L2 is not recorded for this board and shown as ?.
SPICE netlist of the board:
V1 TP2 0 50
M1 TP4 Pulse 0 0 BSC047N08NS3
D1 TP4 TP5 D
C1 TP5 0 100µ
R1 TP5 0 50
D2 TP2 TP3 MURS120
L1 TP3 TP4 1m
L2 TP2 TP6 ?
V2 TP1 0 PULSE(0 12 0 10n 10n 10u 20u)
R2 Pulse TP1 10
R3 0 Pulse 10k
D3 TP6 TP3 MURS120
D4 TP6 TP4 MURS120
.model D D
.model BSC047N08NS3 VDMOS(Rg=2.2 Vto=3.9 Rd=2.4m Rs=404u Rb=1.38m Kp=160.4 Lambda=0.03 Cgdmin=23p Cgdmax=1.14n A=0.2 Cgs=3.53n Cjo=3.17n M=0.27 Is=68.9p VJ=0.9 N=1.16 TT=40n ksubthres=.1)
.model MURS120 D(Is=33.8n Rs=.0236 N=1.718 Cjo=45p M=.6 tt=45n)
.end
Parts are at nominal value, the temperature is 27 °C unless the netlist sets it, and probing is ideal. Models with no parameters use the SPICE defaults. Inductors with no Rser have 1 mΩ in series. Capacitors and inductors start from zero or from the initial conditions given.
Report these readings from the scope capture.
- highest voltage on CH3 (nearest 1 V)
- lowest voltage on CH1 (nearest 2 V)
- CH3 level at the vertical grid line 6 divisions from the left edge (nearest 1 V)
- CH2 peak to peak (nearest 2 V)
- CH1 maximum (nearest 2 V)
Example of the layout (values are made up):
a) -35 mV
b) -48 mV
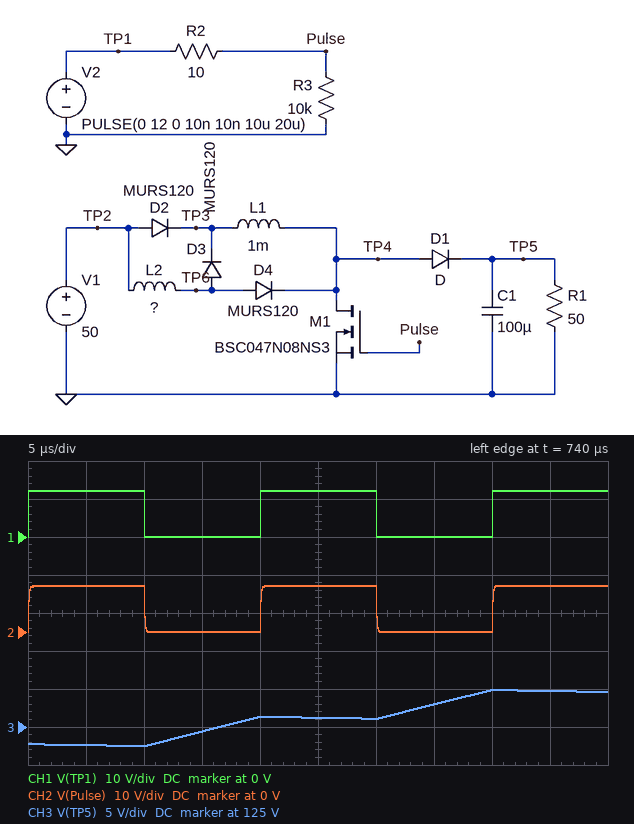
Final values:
a) 130 V
b) 0 V
c) 126 V
d) 12 V
e) 12 V
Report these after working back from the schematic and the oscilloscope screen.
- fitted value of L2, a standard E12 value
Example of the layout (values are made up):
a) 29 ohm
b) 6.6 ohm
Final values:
a) 390 µH
